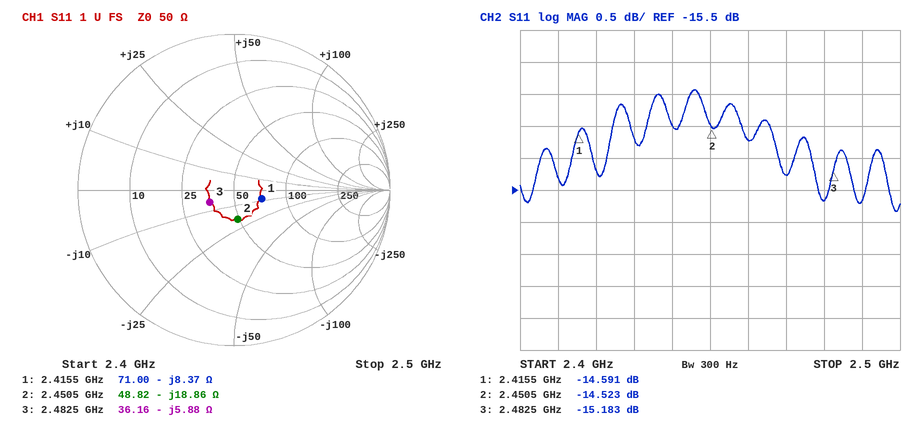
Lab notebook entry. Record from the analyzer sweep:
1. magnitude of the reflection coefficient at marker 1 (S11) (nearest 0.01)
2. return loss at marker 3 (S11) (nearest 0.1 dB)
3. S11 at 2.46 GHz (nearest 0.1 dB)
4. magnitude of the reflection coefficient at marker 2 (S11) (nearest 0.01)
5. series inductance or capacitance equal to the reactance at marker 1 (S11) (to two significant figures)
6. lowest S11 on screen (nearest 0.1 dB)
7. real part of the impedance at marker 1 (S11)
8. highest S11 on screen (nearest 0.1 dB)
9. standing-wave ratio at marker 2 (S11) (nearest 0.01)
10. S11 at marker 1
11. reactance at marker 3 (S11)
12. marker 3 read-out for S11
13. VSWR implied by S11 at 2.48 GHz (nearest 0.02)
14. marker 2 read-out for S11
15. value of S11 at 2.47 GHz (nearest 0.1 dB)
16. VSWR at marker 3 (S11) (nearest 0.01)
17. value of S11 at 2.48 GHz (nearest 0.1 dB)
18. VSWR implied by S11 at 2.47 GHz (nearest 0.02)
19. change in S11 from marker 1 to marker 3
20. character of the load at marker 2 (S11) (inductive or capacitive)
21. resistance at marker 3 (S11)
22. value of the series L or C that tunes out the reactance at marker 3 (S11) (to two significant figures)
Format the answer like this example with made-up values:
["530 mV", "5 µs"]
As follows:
["0.19", "15.2 dB", "-14.7 dB", "0.19", "7.9 pF", "-15.8 dB", "71.00 Ω", "-13.9 dB", "1.46", "-14.591 dB", "-5.88 Ω", "-15.183 dB", "1.40", "-14.523 dB", "-15.3 dB", "1.42", "-15.7 dB", "1.42", "-0.592 dB", "capacitive", "36.16 Ω", "380 pH"]
